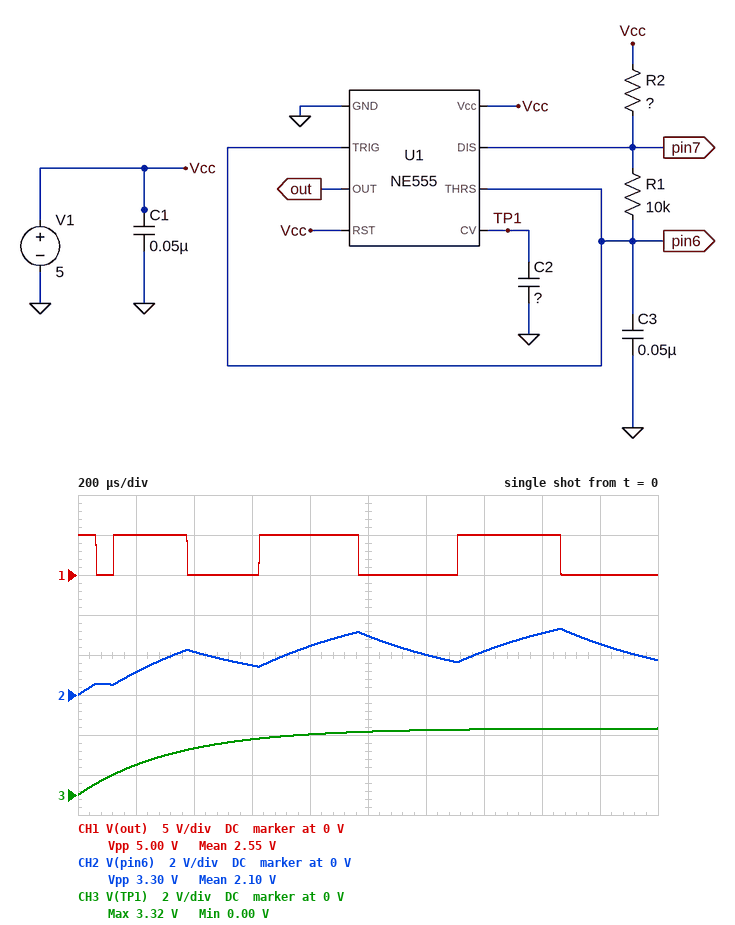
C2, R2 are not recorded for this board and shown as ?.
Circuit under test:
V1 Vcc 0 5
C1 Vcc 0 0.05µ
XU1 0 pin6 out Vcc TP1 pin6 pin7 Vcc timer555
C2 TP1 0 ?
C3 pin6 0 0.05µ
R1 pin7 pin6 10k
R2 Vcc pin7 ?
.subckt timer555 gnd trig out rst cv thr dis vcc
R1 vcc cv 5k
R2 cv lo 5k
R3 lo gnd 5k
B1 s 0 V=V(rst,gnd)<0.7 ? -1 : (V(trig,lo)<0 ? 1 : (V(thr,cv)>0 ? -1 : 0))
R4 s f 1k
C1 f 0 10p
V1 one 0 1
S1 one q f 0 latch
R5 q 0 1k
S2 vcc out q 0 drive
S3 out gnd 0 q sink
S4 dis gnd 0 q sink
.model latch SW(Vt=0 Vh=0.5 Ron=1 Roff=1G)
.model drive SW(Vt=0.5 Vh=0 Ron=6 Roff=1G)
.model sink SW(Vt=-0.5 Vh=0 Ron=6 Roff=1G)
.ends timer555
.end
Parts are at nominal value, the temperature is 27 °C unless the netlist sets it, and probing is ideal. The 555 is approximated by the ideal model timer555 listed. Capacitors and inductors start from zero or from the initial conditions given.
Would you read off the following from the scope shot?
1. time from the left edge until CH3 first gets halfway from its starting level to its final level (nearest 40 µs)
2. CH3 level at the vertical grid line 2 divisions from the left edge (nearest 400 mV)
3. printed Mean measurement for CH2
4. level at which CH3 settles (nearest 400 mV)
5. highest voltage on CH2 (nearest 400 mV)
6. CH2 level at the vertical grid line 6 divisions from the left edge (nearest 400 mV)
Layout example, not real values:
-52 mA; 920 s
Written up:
240 µs; 2.4 V; 2.10 V; 3.2 V; 3.2 V; 2.0 V
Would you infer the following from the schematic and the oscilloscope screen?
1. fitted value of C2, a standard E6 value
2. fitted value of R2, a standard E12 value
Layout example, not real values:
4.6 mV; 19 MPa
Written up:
100 nF; 330 Ω
